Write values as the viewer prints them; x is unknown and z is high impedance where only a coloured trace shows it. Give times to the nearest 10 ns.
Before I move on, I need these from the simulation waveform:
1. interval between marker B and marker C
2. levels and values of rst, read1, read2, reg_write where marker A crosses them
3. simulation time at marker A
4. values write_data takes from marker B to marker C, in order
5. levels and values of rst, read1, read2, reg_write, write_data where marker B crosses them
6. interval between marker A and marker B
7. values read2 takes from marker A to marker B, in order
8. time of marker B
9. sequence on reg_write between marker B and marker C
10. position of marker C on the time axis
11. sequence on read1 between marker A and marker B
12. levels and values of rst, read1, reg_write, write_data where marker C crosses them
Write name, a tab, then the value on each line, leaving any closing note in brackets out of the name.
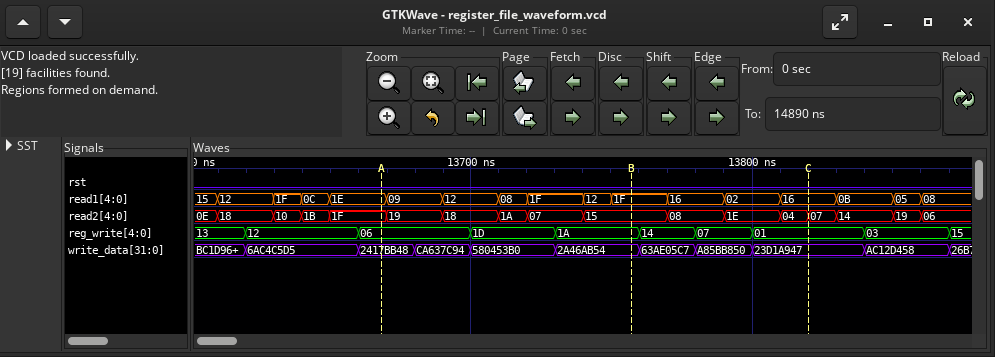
interval between marker B and marker C	60 ns
levels and values of rst, read1, read2, reg_write where marker A crosses them	rst=0, read1=1E, read2=1F, reg_write=06
simulation time at marker A	13670 ns
values write_data takes from marker B to marker C, in order	2A46AB54, 63AE05C7, A85BB850, 23D1A947
levels and values of rst, read1, read2, reg_write, write_data where marker B crosses them	rst=0, read1=1F, read2=15, reg_write=1A, write_data=2A46AB54
interval between marker A and marker B	90 ns
values read2 takes from marker A to marker B, in order	1F, 19, 18, 1A, 07, 15
time of marker B	13760 ns
sequence on reg_write between marker B and marker C	1A, 14, 07, 01
position of marker C on the time axis	13820 ns
sequence on read1 between marker A and marker B	1E, 09, 12, 08, 1F, 12, 1F
levels and values of rst, read1, reg_write, write_data where marker C crosses them	rst=0, read1=16, reg_write=01, write_data=23D1A947
